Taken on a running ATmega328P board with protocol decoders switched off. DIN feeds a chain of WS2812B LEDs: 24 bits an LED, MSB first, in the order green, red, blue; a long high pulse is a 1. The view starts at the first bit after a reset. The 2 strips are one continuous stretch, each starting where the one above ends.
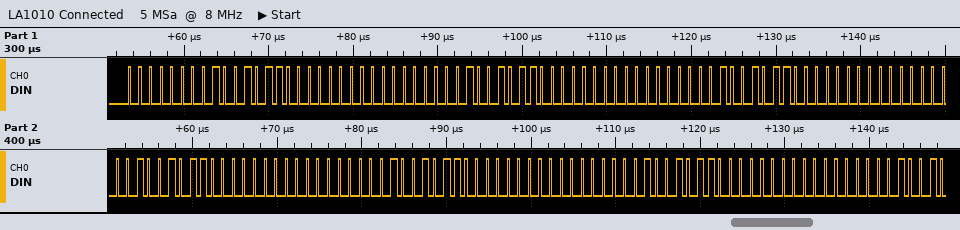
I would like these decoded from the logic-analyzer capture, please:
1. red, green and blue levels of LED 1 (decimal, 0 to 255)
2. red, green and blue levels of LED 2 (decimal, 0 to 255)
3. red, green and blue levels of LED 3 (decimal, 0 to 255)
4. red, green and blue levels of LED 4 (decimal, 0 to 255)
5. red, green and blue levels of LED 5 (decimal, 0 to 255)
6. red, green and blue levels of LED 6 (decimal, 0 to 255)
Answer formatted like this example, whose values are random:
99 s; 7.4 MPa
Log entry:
150, 0, 0; 150, 0, 0; 150, 0, 0; 150, 0, 0; 150, 0, 0; 150, 0, 0
